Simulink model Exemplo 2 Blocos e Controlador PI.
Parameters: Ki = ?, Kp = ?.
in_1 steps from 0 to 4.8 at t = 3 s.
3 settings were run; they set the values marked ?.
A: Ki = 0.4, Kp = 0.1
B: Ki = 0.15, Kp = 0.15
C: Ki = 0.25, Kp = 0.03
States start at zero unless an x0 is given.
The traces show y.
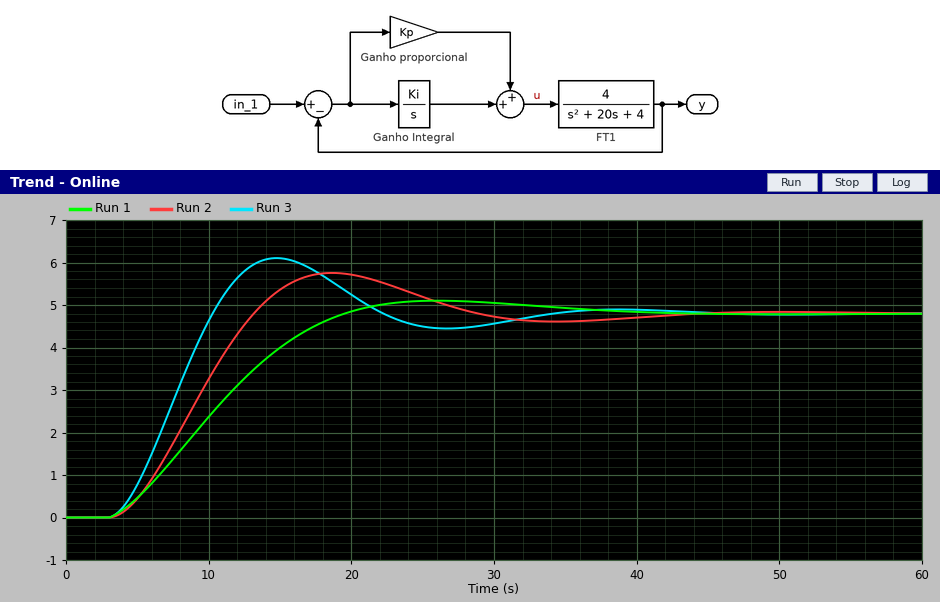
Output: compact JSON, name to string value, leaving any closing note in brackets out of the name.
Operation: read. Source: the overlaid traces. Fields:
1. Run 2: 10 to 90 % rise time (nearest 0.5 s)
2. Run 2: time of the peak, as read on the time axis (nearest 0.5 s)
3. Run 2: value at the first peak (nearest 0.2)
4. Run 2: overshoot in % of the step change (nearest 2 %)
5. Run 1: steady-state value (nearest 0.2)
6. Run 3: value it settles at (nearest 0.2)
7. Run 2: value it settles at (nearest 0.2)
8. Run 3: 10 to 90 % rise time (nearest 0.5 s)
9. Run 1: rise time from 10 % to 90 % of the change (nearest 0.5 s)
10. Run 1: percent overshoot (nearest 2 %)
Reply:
{"Run 2: 10 to 90 % rise time": "7.0 s", "Run 2: time of the peak, as read on the time axis": "18.5 s", "Run 2: value at the first peak": "5.8", "Run 2: overshoot in % of the step change": "20 %", "Run 1: steady-state value": "4.8", "Run 3: value it settles at": "4.8", "Run 2: value it settles at": "4.8", "Run 3: 10 to 90 % rise time": "5.0 s", "Run 1: rise time from 10 % to 90 % of the change": "11.5 s", "Run 1: percent overshoot": "6 %"}
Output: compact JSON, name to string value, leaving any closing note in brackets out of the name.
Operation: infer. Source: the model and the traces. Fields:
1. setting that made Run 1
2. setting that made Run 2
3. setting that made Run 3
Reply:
{"setting that made Run 1": "B", "setting that made Run 2": "C", "setting that made Run 3": "A"}
